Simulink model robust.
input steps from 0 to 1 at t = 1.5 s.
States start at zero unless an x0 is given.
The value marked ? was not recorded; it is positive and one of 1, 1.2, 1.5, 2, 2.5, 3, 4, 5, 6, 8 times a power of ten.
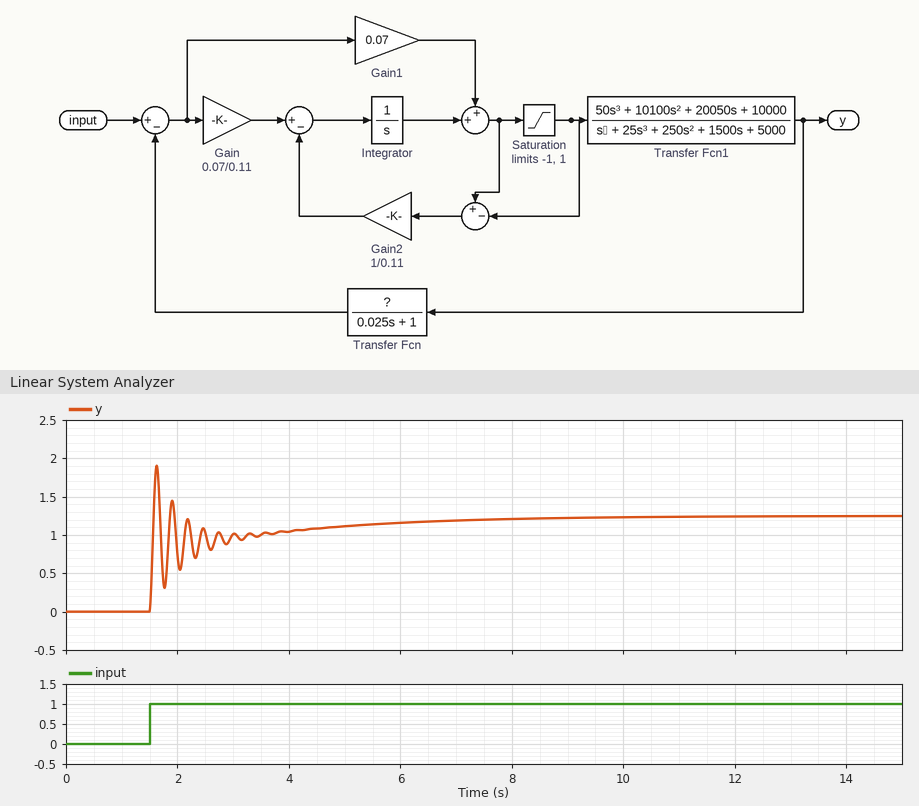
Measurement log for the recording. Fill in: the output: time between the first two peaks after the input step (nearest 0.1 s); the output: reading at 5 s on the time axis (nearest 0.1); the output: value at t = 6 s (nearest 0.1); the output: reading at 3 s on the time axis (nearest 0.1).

0.3 s
1.1
1.2
1.0
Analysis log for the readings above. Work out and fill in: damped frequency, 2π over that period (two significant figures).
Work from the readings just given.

21 rad/s
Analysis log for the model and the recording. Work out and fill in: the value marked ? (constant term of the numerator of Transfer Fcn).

0.8
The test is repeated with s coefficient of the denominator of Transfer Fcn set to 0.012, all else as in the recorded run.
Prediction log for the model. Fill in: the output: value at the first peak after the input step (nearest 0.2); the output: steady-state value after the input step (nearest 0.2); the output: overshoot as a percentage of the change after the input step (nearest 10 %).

1.6
1.2
30 %
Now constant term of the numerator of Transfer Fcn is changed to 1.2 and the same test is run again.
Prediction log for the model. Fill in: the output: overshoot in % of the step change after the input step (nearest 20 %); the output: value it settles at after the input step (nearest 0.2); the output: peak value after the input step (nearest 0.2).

80 %
0.8
1.4
